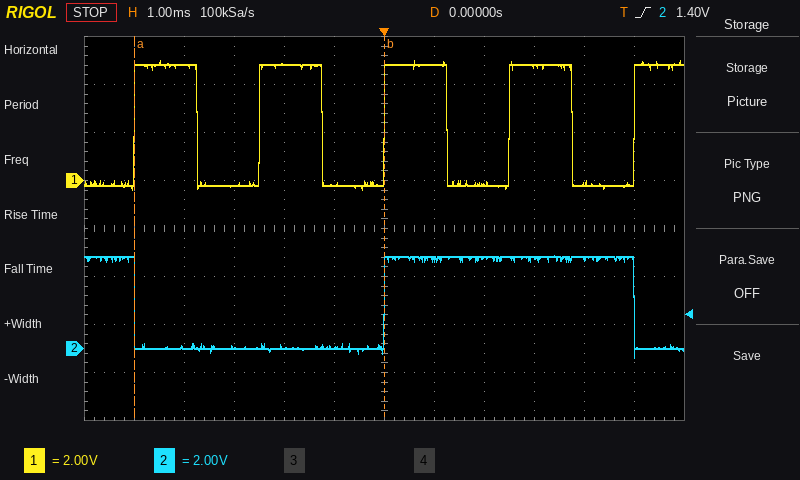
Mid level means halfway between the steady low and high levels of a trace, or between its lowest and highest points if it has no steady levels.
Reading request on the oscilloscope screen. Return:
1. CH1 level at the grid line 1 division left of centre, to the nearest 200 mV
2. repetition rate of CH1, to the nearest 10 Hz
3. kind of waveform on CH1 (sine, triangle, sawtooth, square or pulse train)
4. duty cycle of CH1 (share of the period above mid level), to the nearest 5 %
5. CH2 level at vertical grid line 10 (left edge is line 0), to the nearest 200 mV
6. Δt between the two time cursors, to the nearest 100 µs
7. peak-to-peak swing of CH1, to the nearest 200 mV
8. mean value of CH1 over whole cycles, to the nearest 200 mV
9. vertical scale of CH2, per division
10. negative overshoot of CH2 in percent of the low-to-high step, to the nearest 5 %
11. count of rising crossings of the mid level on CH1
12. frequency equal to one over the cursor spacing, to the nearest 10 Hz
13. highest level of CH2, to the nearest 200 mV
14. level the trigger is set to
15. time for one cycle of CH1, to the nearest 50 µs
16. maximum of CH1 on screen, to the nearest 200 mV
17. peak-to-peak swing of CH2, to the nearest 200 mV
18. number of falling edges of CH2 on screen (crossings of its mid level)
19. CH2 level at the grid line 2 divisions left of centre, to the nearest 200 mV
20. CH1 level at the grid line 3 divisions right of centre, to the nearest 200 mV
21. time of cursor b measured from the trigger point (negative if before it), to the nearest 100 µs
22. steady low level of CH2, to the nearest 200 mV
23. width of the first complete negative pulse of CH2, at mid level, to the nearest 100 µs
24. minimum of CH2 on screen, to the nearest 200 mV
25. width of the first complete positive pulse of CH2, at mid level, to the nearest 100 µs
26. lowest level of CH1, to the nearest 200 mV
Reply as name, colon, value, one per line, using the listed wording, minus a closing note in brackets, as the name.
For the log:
CH1 level at the grid line 1 division left of centre, to the nearest 200 mV: -200 mV
repetition rate of CH1, to the nearest 10 Hz: 400 Hz
kind of waveform on CH1: square
duty cycle of CH1 (share of the period above mid level), to the nearest 5 %: 50 %
CH2 level at vertical grid line 10 (left edge is line 0), to the nearest 200 mV: 3.8 V
Δt between the two time cursors, to the nearest 100 µs: 5.0 ms
peak-to-peak swing of CH1, to the nearest 200 mV: 5.4 V
mean value of CH1 over whole cycles, to the nearest 200 mV: 2.4 V
vertical scale of CH2, per division: 2 V
negative overshoot of CH2 in percent of the low-to-high step, to the nearest 5 %: 10 %
count of rising crossings of the mid level on CH1: 5
frequency equal to one over the cursor spacing, to the nearest 10 Hz: 200 Hz
highest level of CH2, to the nearest 200 mV: 3.8 V
level the trigger is set to: 1.40 V
time for one cycle of CH1, to the nearest 50 µs: 2.50 ms
maximum of CH1 on screen, to the nearest 200 mV: 5.0 V
peak-to-peak swing of CH2, to the nearest 200 mV: 4.2 V
number of falling edges of CH2 on screen: 2
CH2 level at the grid line 2 divisions left of centre, to the nearest 200 mV: 0.0 V
CH1 level at the grid line 3 divisions right of centre, to the nearest 200 mV: 4.8 V
time of cursor b measured from the trigger point (negative if before it), to the nearest 100 µs: 0.0 ms
steady low level of CH2, to the nearest 200 mV: 0.0 V
width of the first complete negative pulse of CH2, at mid level, to the nearest 100 µs: 5.0 ms
minimum of CH2 on screen, to the nearest 200 mV: -400 mV
width of the first complete positive pulse of CH2, at mid level, to the nearest 100 µs: 5.0 ms
lowest level of CH1, to the nearest 200 mV: -400 mV
